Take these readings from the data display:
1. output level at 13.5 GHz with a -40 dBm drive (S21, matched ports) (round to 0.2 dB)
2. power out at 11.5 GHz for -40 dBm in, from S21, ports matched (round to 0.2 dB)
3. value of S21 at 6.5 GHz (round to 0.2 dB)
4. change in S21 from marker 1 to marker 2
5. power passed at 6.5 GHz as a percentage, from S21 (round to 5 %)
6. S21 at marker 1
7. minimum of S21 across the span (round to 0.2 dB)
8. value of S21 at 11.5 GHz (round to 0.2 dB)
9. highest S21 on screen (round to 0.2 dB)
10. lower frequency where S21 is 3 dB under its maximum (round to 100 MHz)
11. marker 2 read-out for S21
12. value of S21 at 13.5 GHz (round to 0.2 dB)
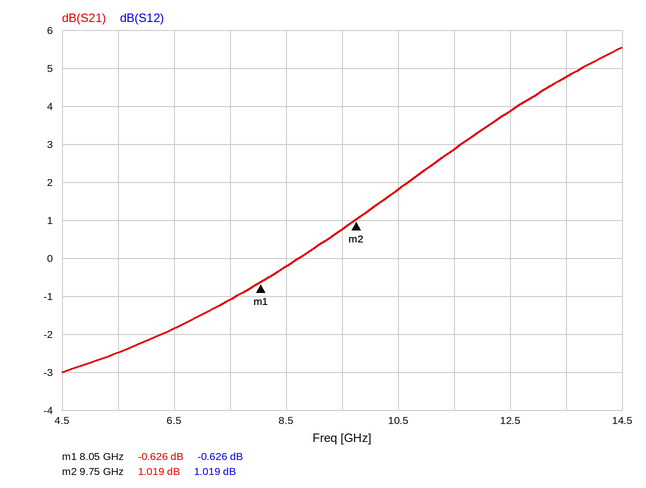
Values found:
-35.2 dBm
-37.2 dBm
-1.8 dB
1.645 dB
65 %
-0.626 dB
-3.0 dB
2.8 dB
5.6 dB
11.2 GHz
1.019 dB
4.8 dB
